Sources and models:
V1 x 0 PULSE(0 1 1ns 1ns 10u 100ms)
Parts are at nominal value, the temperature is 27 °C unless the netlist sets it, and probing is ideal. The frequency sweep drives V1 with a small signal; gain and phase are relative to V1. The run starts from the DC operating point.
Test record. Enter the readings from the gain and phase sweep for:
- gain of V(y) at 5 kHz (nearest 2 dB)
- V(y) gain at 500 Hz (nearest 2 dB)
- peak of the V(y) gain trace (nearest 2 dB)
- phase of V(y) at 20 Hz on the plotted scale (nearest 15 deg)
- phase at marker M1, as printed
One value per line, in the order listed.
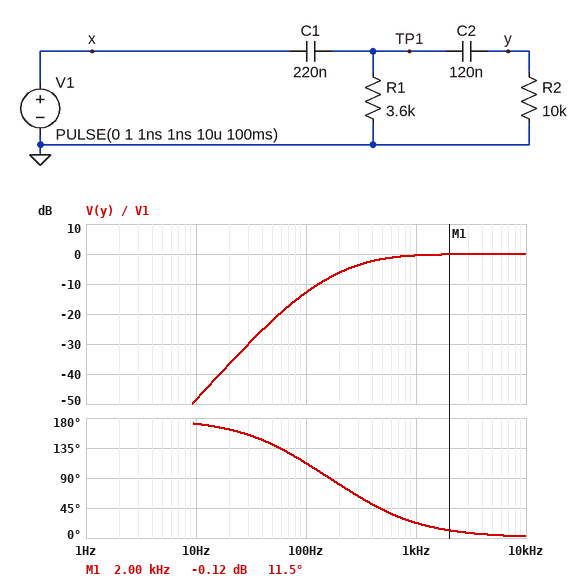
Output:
0 dB
-2 dB
0 dB
165 deg
11.5 deg
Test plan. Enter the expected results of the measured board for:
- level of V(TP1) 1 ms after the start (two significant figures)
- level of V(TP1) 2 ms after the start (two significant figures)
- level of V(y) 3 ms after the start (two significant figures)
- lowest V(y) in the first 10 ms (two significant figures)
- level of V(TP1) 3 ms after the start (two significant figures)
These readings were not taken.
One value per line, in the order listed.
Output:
230 mV
88 mV
-69 mV
-100 mV
46 mV
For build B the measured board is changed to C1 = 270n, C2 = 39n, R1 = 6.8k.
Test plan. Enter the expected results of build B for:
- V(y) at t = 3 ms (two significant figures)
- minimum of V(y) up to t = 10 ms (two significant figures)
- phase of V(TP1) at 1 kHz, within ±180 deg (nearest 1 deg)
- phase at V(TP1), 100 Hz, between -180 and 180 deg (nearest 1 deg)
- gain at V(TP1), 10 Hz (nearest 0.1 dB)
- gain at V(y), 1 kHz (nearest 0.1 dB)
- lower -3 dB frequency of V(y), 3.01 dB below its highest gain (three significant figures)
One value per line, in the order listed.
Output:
-45 mV
-78 mV
8 deg
38 deg
-18.8 dB
-0.9 dB
491 Hz
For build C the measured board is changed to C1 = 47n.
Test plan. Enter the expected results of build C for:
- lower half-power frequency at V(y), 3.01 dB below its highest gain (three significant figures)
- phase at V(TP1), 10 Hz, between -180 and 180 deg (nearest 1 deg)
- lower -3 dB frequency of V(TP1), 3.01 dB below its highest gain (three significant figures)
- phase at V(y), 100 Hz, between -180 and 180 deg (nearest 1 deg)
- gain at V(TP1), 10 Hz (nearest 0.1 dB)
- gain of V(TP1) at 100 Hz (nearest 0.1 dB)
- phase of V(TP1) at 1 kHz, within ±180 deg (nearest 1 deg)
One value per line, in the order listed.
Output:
1.32 kHz
88 deg
1.31 kHz
129 deg
-39.5 dB
-20.8 dB
51 deg
